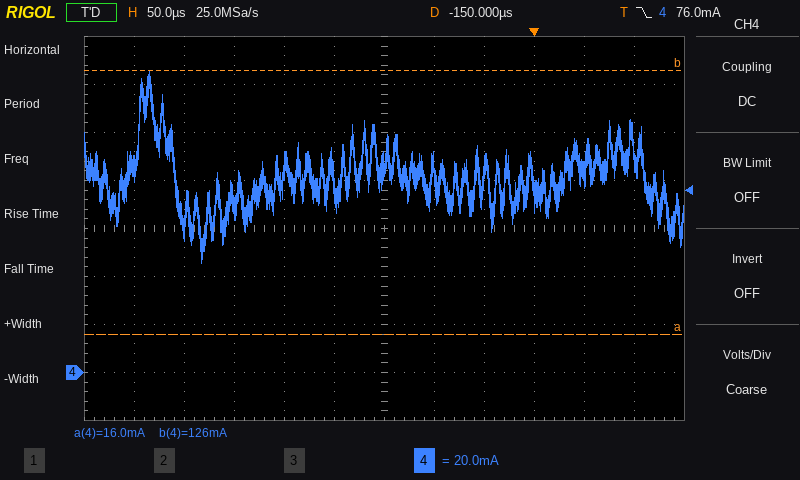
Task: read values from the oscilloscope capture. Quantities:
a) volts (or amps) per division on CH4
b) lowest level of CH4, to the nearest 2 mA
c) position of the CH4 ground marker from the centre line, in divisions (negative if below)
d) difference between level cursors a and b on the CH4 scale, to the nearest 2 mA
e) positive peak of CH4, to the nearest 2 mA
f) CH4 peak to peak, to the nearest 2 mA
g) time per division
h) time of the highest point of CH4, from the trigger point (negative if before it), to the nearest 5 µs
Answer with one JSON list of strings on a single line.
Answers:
["20 mA", "46 mA", "-3.0 div", "110 mA", "126 mA", "80 mA", "50 µs", "-385 µs"]
